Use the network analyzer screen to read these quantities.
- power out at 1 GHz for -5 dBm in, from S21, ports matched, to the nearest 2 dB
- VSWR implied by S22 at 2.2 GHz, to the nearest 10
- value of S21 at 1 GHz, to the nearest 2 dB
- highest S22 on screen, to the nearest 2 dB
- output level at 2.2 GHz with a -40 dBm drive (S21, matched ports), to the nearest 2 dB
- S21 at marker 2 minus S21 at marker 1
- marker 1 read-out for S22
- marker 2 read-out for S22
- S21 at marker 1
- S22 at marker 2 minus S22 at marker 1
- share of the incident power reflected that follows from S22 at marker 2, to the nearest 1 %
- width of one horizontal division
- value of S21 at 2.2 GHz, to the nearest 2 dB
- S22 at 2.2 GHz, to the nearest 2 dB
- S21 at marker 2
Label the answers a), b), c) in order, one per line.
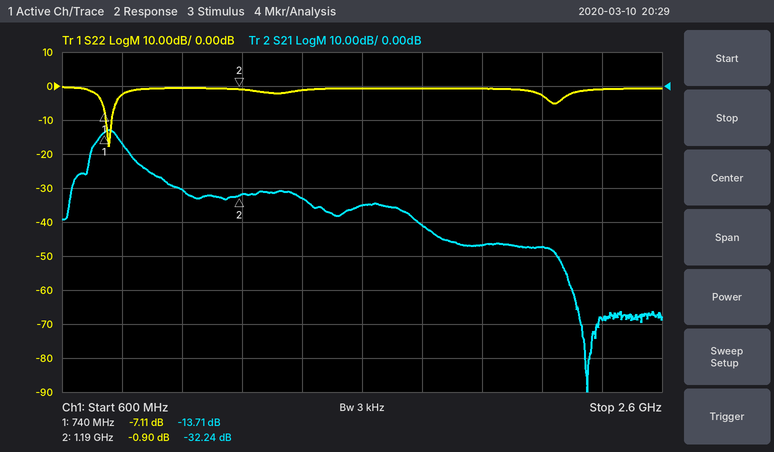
a) -36 dBm
b) 10
c) -30 dB
d) 0 dB
e) -88 dBm
f) -18.53 dB
g) -7.11 dB
h) -0.90 dB
i) -13.71 dB
j) 6.21 dB
k) 81 %
l) 200 MHz
m) -48 dB
n) -2 dB
o) -32.24 dB
